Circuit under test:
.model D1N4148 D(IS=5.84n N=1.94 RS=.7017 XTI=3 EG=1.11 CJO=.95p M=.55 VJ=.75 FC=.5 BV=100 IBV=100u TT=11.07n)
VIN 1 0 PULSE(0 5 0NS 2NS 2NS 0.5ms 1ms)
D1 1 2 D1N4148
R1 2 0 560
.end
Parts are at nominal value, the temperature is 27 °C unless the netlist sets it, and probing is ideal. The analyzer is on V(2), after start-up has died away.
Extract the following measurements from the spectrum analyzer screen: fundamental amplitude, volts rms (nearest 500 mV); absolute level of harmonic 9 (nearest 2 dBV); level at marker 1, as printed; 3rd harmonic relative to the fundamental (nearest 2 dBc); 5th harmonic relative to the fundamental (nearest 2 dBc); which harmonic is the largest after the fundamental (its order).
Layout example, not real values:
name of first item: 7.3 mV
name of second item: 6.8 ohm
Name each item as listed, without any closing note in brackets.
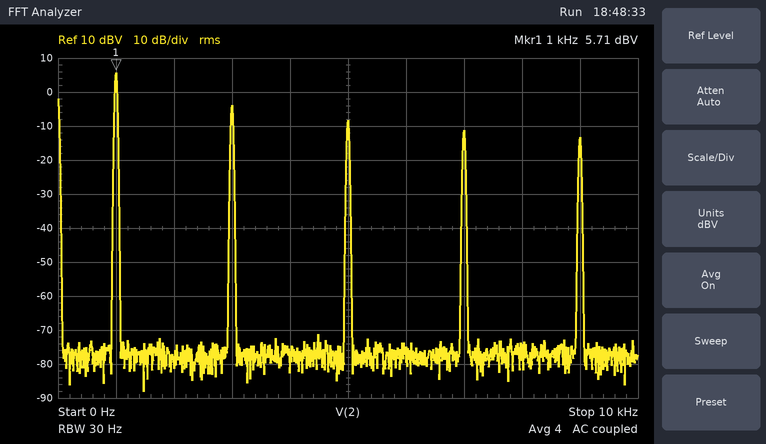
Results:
fundamental amplitude, volts rms: 2.0 V
absolute level of harmonic 9: -14 dBV
level at marker 1, as printed: 5.71 dBV
3rd harmonic relative to the fundamental: -10 dBc
5th harmonic relative to the fundamental: -14 dBc
which harmonic is the largest after the fundamental: 3
